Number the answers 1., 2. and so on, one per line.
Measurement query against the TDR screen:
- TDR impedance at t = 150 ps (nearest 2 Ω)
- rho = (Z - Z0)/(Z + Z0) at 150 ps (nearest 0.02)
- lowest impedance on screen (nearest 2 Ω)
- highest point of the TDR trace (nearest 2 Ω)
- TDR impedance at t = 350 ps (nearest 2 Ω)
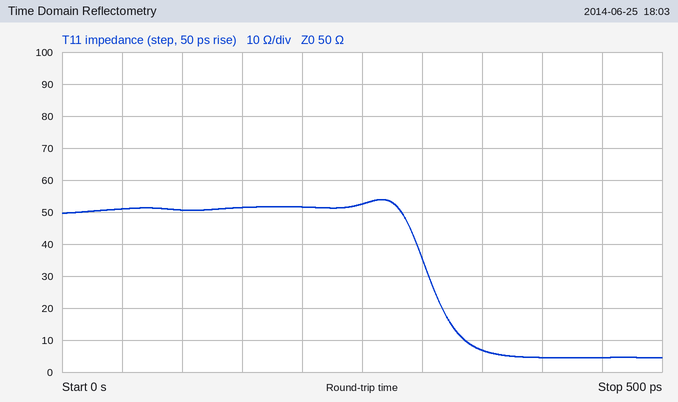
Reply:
1. 52 Ω
2. +0.02
3. 4 Ω
4. 54 Ω
5. 6 Ω
